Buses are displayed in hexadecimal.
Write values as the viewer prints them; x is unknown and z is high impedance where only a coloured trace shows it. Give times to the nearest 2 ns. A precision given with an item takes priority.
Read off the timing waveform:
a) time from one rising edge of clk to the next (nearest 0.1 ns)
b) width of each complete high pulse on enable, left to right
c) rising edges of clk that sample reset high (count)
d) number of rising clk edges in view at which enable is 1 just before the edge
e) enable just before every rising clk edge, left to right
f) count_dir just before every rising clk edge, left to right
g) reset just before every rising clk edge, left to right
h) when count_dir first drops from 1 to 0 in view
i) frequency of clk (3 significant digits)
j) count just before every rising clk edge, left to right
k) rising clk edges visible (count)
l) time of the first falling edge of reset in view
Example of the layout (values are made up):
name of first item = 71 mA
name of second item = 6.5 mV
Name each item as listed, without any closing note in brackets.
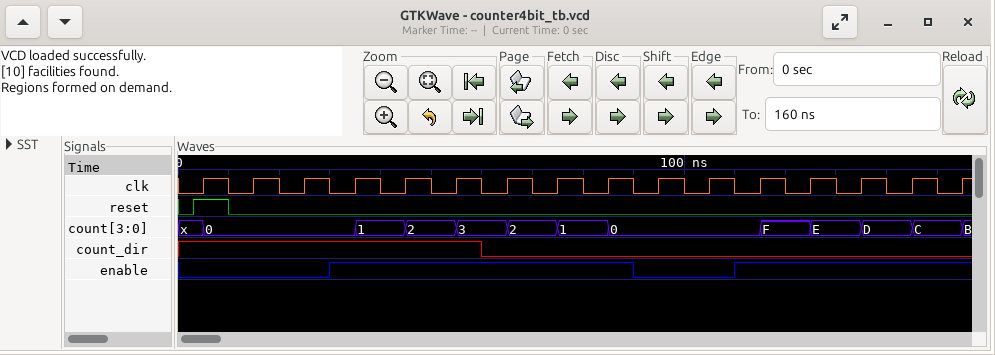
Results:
time from one rising edge of clk to the next = 10 ns
width of each complete high pulse on enable, left to right = 60 ns
rising edges of clk that sample reset high = 1
number of rising clk edges in view at which enable is 1 just before the edge = 11
enable just before every rising clk edge, left to right = 0 0 0 1 1 1 1 1 1 0 0 1 1 1 1 1
count_dir just before every rising clk edge, left to right = 1 1 1 1 1 1 0 0 0 0 0 0 0 0 0 0
reset just before every rising clk edge, left to right = 1 0 0 0 0 0 0 0 0 0 0 0 0 0 0 0
when count_dir first drops from 1 to 0 in view = 60 ns
frequency of clk = 100 MHz
count just before every rising clk edge, left to right = x, 0, 0, 0, 1, 2, 3, 2, 1, 0, 0, 0, F, E, D, C
rising clk edges visible = 16
time of the first falling edge of reset in view = 10 ns
